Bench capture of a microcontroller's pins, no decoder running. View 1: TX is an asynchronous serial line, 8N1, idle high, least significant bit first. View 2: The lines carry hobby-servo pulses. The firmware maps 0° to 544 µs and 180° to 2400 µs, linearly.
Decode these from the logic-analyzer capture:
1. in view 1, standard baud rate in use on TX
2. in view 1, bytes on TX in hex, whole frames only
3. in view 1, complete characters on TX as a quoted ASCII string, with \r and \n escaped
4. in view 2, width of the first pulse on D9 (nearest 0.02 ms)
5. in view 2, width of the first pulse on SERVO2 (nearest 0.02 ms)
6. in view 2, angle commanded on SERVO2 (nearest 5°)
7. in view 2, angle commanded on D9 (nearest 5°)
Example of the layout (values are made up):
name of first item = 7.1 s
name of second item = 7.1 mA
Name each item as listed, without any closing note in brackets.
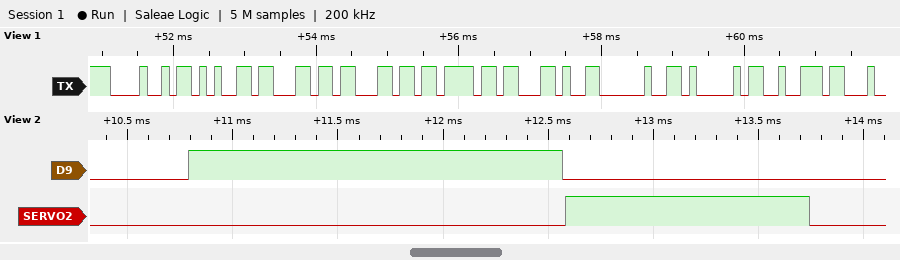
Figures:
in view 1, standard baud rate in use on TX = 9600 baud
in view 1, bytes on TX in hex, whole frames only = 48 65 6C 6C 6F 2C 20 41 72
in view 1, complete characters on TX as a quoted ASCII string, with \r and \n escaped = "Hello, Ar"
in view 2, width of the first pulse on D9 = 1.78 ms
in view 2, width of the first pulse on SERVO2 = 1.16 ms
in view 2, angle commanded on SERVO2 = 60°
in view 2, angle commanded on D9 = 120°
